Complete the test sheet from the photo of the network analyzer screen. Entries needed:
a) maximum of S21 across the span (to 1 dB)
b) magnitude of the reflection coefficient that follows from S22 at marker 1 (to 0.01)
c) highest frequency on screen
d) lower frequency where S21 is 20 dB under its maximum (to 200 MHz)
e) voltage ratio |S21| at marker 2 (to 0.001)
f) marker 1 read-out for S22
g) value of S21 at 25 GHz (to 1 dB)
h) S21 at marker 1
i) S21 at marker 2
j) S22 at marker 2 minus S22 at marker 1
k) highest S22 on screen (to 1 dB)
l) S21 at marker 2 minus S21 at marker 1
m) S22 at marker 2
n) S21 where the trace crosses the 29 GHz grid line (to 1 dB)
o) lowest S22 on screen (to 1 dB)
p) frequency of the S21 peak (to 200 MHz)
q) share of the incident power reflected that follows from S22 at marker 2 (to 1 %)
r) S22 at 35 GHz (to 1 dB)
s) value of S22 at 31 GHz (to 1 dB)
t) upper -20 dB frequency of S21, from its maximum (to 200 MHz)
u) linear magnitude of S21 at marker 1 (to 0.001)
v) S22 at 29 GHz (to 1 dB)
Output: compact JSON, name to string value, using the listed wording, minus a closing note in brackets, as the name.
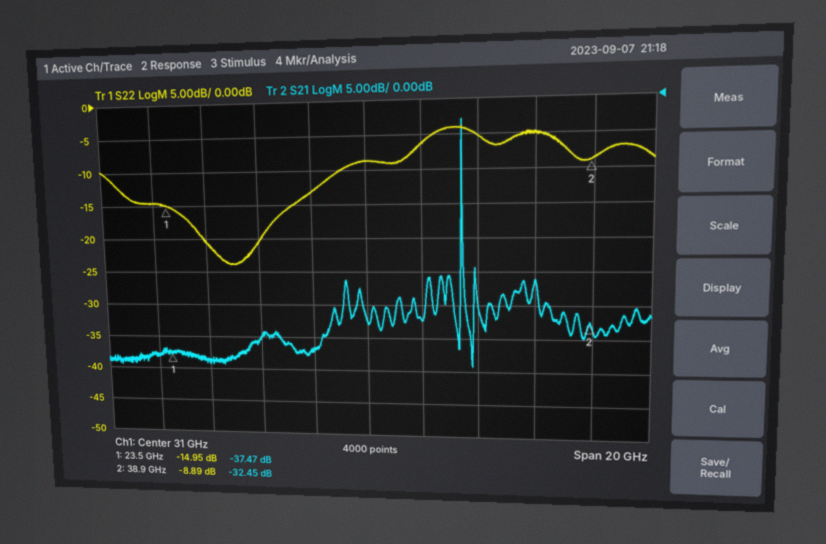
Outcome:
{"maximum of S21 across the span": "-3 dB", "magnitude of the reflection coefficient that follows from S22 at marker 1": "0.18", "highest frequency on screen": "41 GHz", "lower frequency where S21 is 20 dB under its maximum": "34.4 GHz", "voltage ratio |S21| at marker 2": "0.024", "marker 1 read-out for S22": "-14.95 dB", "value of S21 at 25 GHz": "-39 dB", "S21 at marker 1": "-37.47 dB", "S21 at marker 2": "-32.45 dB", "S22 at marker 2 minus S22 at marker 1": "6.06 dB", "highest S22 on screen": "-4 dB", "S21 at marker 2 minus S21 at marker 1": "5.02 dB", "S22 at marker 2": "-8.89 dB", "S21 where the trace crosses the 29 GHz grid line": "-37 dB", "lowest S22 on screen": "-24 dB", "frequency of the S21 peak": "34.4 GHz", "share of the incident power reflected that follows from S22 at marker 2": "13 %", "S22 at 35 GHz": "-5 dB", "value of S22 at 31 GHz": "-9 dB", "upper -20 dB frequency of S21, from its maximum": "34.4 GHz", "linear magnitude of S21 at marker 1": "0.013", "S22 at 29 GHz": "-13 dB"}
